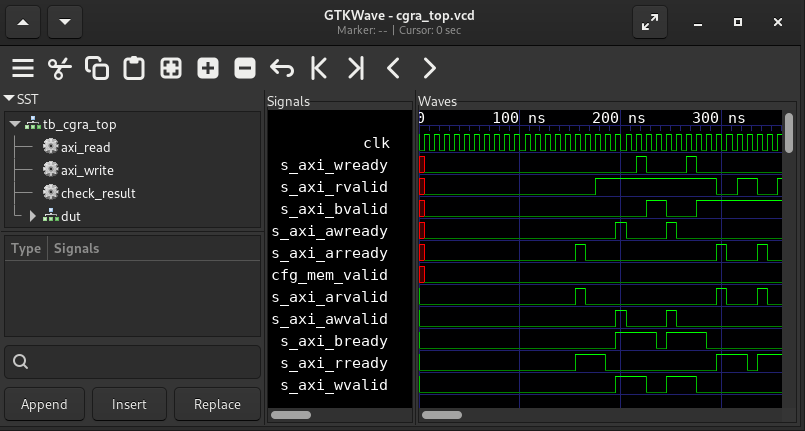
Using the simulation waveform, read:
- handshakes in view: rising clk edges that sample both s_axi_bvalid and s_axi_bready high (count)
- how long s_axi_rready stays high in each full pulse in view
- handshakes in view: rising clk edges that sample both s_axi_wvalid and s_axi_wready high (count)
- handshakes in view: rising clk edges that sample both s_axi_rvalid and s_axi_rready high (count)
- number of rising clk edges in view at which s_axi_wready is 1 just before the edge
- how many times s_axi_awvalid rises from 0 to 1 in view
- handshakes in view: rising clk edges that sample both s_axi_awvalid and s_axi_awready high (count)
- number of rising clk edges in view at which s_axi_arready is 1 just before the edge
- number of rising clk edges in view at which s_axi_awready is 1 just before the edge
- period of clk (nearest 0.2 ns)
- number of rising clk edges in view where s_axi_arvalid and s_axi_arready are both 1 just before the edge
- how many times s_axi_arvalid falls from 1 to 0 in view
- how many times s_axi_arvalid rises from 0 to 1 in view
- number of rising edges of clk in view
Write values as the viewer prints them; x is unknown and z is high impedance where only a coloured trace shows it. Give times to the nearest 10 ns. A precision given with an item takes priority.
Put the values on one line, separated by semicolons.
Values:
2; 30 ns, 30 ns; 2; 2; 2; 2; 2; 3; 2; 10 ns; 3; 3; 3; 36
